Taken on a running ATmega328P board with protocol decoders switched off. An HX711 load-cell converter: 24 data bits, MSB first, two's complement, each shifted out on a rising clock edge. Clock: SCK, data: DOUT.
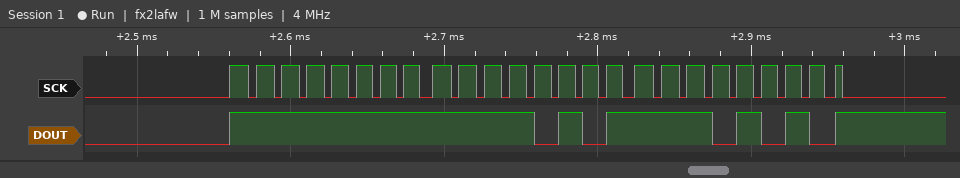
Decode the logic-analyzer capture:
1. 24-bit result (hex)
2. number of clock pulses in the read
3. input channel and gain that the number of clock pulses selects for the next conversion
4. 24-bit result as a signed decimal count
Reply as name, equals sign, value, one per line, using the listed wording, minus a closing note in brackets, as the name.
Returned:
24-bit result = 0xFFF5EA
number of clock pulses in the read = 25
input channel and gain that the number of clock pulses selects for the next conversion = channel A, gain 128
24-bit result as a signed decimal count = -2582
